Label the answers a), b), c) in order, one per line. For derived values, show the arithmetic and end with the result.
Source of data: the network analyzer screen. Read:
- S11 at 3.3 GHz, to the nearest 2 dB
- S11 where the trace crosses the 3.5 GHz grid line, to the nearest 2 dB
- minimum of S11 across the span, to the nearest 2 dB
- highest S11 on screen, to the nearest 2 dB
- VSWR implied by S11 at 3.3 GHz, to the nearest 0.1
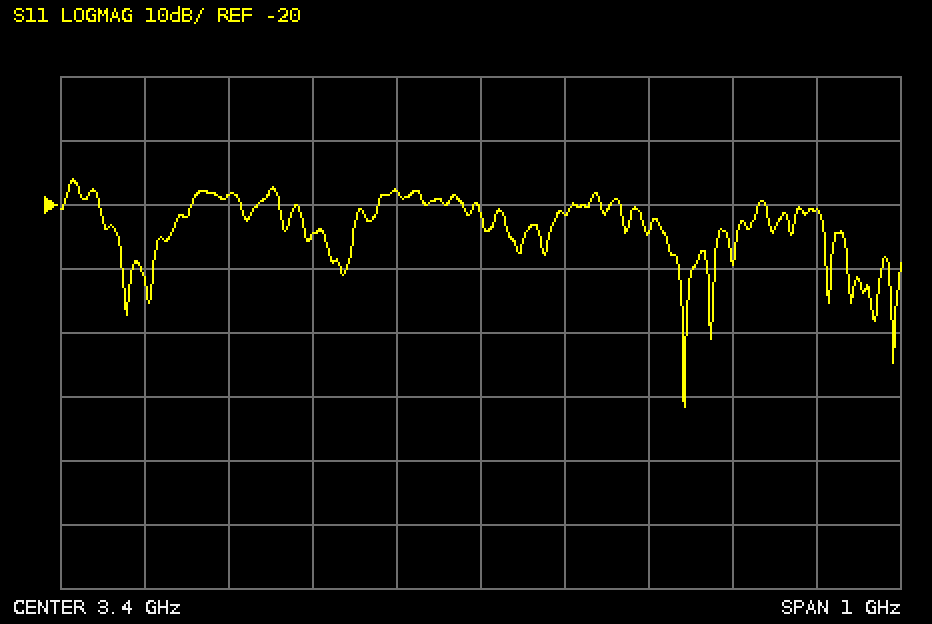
a) -18 dB
b) -22 dB
c) -52 dB
d) -16 dB
e) |Γ| = 10^(-18/20) = 0.1259; VSWR = (1 + 0.1259)/(1 − 0.1259) ≈ 1.3
